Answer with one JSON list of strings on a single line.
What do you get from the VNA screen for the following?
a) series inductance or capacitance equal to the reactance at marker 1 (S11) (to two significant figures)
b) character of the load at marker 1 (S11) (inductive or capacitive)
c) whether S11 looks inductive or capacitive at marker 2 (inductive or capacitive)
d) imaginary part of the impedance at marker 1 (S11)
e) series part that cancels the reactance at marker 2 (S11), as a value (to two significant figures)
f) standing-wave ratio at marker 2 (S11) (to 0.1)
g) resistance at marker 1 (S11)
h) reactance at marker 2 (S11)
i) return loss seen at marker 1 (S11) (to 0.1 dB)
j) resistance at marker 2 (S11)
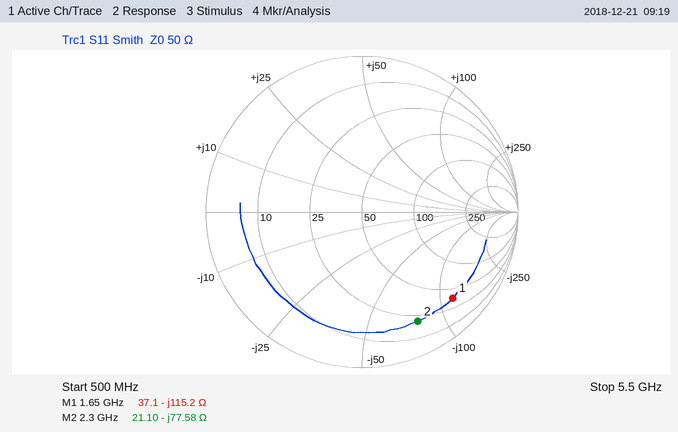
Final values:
["840 fF", "capacitive", "capacitive", "-115.2 Ω", "5.4 nH", "8.4", "37.1 Ω", "-77.58 Ω", "1.9 dB", "21.10 Ω"]
